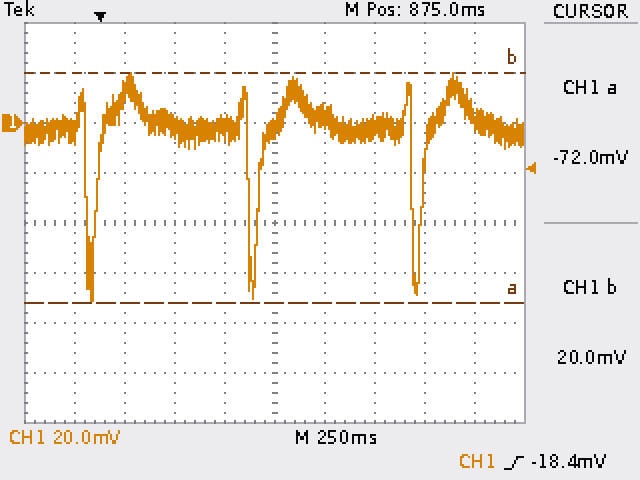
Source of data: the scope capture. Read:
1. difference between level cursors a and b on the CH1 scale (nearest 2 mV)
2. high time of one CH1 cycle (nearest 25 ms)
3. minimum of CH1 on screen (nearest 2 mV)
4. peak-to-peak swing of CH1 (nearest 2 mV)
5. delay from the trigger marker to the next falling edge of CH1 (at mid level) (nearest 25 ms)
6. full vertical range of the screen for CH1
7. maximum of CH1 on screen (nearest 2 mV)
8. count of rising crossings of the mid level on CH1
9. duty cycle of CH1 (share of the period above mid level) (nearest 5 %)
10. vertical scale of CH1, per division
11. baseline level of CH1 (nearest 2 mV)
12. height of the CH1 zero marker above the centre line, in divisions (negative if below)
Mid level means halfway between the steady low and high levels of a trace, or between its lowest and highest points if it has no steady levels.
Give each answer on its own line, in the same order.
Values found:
92 mV
750 ms
-72 mV
92 mV
750 ms
160 mV
20 mV
3
95 %
20 mV
-2 mV
+2.0 div
